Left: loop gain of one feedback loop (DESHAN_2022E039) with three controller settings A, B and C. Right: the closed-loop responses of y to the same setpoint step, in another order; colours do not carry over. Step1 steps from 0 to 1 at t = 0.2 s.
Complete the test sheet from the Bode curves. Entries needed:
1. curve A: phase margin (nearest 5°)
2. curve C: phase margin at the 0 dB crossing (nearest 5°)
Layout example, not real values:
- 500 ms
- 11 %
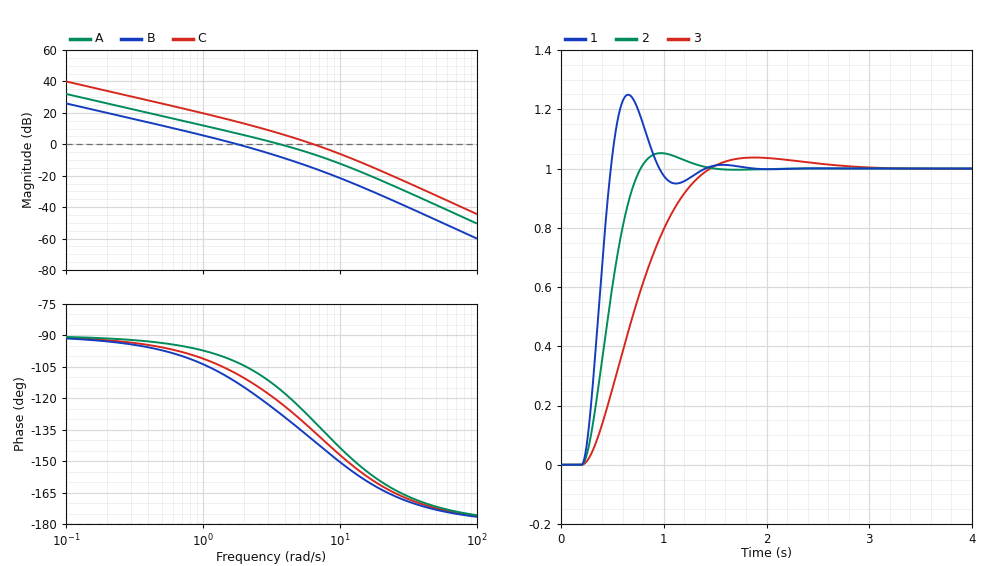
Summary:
- 65°
- 45°
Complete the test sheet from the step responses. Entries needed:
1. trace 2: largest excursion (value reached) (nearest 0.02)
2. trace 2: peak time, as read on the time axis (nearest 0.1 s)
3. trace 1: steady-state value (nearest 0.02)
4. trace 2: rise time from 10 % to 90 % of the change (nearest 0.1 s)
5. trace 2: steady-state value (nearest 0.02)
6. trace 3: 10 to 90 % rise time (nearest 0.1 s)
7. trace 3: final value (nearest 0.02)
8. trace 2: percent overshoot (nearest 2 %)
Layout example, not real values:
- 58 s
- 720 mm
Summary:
- 1.06
- 1.0 s
- 1.00
- 0.4 s
- 1.00
- 0.8 s
- 1.00
- 6 %
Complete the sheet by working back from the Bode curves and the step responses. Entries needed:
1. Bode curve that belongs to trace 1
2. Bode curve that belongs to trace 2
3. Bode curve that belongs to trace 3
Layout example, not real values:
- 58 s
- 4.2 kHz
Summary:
- C
- A
- B
